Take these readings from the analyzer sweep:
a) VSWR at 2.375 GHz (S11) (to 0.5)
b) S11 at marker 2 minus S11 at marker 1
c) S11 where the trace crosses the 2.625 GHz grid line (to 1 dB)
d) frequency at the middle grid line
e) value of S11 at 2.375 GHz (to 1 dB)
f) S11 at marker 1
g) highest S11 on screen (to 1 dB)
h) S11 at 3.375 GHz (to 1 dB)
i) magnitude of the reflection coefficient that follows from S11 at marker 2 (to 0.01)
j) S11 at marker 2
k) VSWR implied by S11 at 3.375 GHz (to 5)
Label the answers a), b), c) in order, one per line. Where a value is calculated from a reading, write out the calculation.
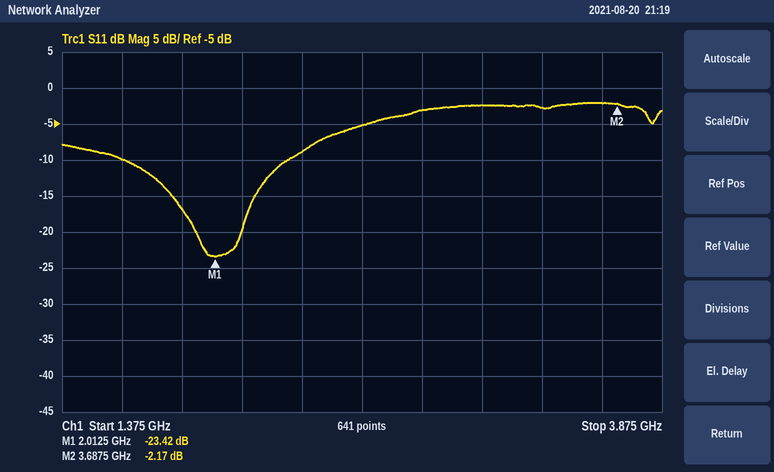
a) |Γ| = 10^(-9/20) = 0.3548; VSWR = (1 + 0.3548)/(1 − 0.3548) ≈ 2.10, so 2.0 to the nearest 0.5
b) -2.17 − (-23.42) = 21.25 dB
c) -5 dB
d) 2.625 GHz
e) -9 dB
f) -23.42 dB
g) -2 dB
h) -3 dB
i) 10^(-2.17/20) ≈ 0.78
j) -2.17 dB
k) |Γ| = 10^(-3/20) = 0.7079; VSWR = (1 + 0.7079)/(1 − 0.7079) ≈ 5.85, so 5 to the nearest 5
